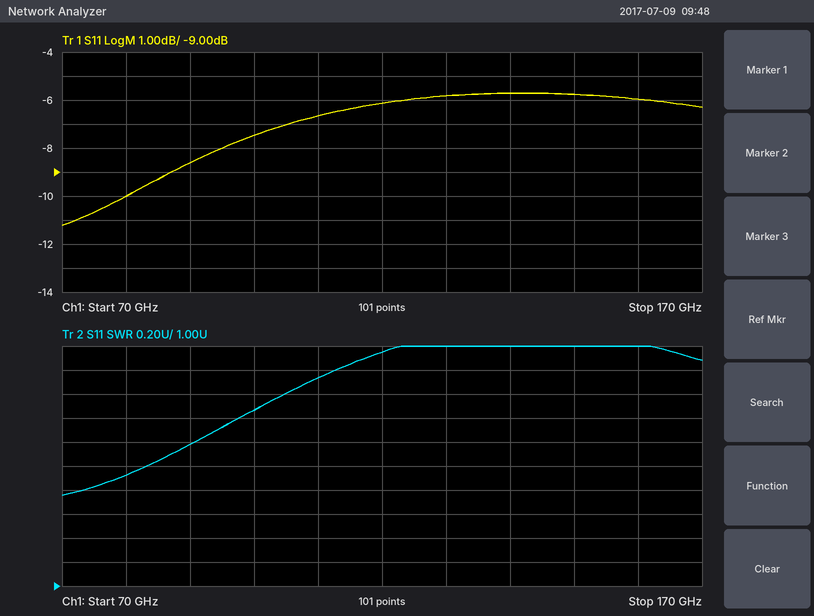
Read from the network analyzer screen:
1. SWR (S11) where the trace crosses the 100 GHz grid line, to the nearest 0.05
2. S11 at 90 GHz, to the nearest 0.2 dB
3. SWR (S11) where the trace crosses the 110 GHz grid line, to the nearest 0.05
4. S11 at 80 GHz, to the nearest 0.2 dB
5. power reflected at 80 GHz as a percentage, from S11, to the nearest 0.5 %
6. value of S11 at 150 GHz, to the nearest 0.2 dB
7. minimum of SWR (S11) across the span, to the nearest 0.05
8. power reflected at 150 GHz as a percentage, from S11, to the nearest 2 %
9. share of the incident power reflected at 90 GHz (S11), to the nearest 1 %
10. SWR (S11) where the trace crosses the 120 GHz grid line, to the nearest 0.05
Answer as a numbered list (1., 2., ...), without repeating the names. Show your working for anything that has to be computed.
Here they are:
1. 2.45
2. -8.6 dB
3. 2.75
4. -10.0 dB
5. 10^(-10/10) ≈ 10.0 %
6. -5.8 dB
7. 1.75
8. 10^(-5.8/10) ≈ 26 %
9. 10^(-8.6/10) ≈ 14 %
10. 2.95
